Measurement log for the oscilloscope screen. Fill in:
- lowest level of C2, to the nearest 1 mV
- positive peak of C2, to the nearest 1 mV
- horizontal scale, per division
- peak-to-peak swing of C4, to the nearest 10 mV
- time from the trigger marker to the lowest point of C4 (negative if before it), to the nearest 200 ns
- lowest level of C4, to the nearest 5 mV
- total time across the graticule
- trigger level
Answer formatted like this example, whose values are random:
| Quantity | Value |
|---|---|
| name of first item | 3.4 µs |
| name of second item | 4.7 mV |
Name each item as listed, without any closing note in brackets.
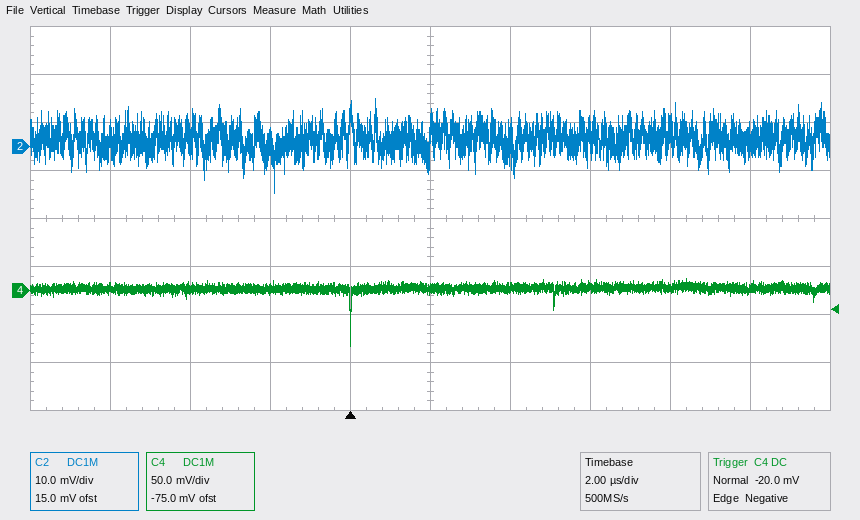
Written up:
| Quantity | Value |
|---|---|
| lowest level of C2, to the nearest 1 mV | -10 mV |
| positive peak of C2, to the nearest 1 mV | 10 mV |
| horizontal scale, per division | 2 µs |
| peak-to-peak swing of C4, to the nearest 10 mV | 70 mV |
| time from the trigger marker to the lowest point of C4 (negative if before it), to the nearest 200 ns | 0.0 µs |
| lowest level of C4, to the nearest 5 mV | -55 mV |
| total time across the graticule | 20 µs |
| trigger level | -20.0 mV |
